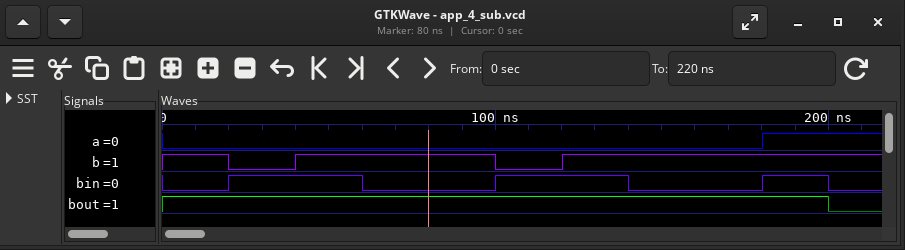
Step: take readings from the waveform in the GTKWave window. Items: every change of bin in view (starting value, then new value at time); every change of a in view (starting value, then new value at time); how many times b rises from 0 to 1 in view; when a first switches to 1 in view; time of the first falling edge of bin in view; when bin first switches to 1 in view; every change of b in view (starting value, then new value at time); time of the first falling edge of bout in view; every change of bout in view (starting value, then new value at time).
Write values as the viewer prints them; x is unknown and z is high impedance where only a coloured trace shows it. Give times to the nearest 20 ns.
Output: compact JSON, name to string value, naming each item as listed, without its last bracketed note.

{"every change of bin in view": "0, 1 at 20 ns, 0 at 60 ns, 1 at 100 ns, 0 at 140 ns, 1 at 180 ns, 0 at 200 ns", "every change of a in view": "0, 1 at 180 ns", "how many times b rises from 0 to 1 in view": "2", "when a first switches to 1 in view": "180 ns", "time of the first falling edge of bin in view": "60 ns", "when bin first switches to 1 in view": "20 ns", "every change of b in view": "1, 0 at 20 ns, 1 at 40 ns, 0 at 100 ns, 1 at 120 ns", "time of the first falling edge of bout in view": "200 ns", "every change of bout in view": "1, 0 at 200 ns"}
